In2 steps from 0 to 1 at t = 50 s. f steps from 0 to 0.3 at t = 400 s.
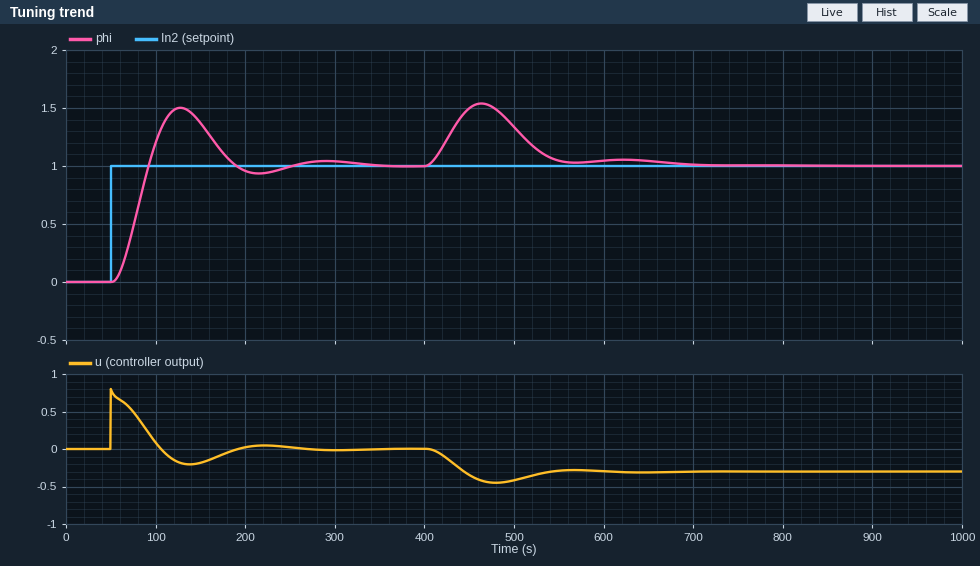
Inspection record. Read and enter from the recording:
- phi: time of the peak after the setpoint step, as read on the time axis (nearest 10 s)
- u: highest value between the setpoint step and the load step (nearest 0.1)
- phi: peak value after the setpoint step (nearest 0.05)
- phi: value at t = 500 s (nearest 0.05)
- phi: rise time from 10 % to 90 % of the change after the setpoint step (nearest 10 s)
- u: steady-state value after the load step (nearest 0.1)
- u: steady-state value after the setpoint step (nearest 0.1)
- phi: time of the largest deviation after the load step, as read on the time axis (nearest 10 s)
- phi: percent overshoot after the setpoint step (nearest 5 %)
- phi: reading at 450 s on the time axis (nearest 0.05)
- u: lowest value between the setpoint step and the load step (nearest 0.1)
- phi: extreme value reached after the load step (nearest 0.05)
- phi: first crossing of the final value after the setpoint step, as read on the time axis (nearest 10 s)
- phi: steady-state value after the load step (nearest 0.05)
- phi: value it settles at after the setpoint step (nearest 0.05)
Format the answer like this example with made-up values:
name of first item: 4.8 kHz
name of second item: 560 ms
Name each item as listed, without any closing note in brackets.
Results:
phi: time of the peak after the setpoint step, as read on the time axis: 130 s
u: highest value between the setpoint step and the load step: 0.8
phi: peak value after the setpoint step: 1.50
phi: value at t = 500 s: 1.35
phi: rise time from 10 % to 90 % of the change after the setpoint step: 30 s
u: steady-state value after the load step: -0.3
u: steady-state value after the setpoint step: 0.0
phi: time of the largest deviation after the load step, as read on the time axis: 460 s
phi: percent overshoot after the setpoint step: 50 %
phi: reading at 450 s on the time axis: 1.50
u: lowest value between the setpoint step and the load step: -0.2
phi: extreme value reached after the load step: 1.55
phi: first crossing of the final value after the setpoint step, as read on the time axis: 90 s
phi: steady-state value after the load step: 1.00
phi: value it settles at after the setpoint step: 1.00
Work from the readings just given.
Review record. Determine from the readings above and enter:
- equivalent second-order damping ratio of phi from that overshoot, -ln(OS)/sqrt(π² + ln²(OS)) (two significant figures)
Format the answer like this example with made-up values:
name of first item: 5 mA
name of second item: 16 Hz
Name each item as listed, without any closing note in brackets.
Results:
equivalent second-order damping ratio of phi from that overshoot, -ln(OS)/sqrt(π² + ln²(OS)): 0.22
